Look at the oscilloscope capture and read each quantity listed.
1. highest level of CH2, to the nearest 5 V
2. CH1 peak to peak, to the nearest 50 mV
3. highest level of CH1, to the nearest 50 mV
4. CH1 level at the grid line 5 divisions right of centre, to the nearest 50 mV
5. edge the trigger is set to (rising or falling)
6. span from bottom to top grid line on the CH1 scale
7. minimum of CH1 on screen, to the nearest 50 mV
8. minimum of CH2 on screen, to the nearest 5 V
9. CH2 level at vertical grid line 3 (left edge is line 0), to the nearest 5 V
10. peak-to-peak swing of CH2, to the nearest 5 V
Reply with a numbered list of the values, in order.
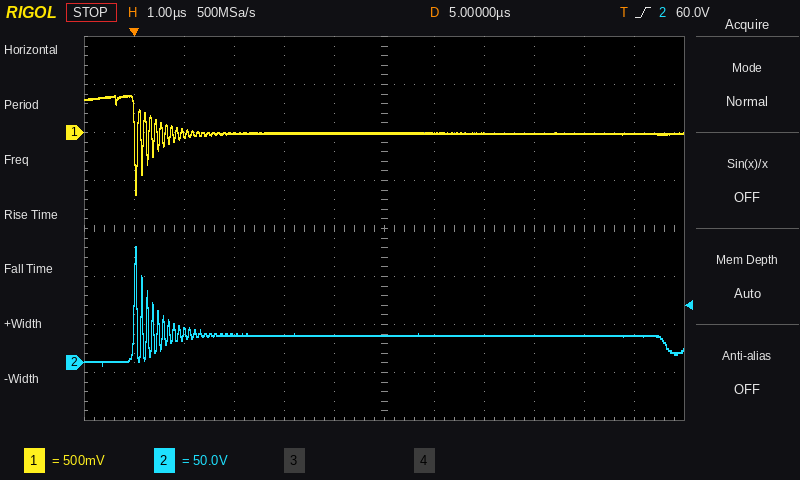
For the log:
1. 120 V
2. 1.05 V
3. 400 mV
4. 0 mV
5. rising
6. 4 V
7. -650 mV
8. -5 V
9. 30 V
10. 125 V
